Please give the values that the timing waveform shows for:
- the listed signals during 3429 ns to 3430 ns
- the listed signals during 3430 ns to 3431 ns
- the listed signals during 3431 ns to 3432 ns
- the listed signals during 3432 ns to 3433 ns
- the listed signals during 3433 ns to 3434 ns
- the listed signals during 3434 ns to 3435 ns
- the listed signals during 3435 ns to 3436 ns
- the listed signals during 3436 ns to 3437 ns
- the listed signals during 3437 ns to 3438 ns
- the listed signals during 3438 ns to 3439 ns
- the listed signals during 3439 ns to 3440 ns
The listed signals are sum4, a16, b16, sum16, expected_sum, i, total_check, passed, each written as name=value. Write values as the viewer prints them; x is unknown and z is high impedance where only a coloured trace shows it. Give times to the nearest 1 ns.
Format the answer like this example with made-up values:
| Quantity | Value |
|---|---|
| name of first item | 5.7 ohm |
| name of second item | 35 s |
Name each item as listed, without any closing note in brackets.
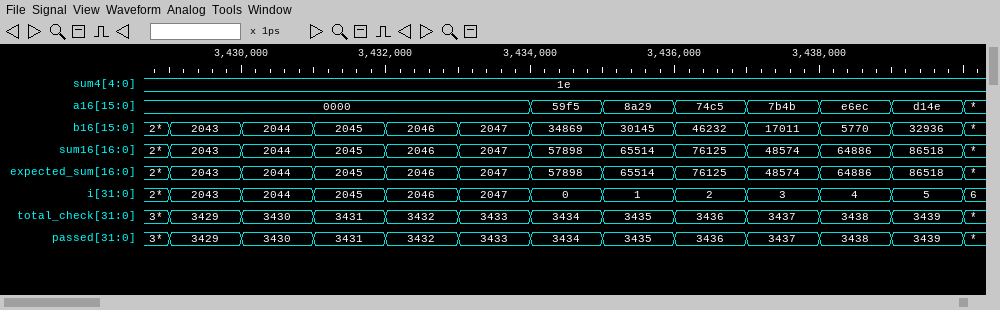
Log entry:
| Quantity | Value |
|---|---|
| the listed signals during 3429 ns to 3430 ns | sum4=1e, a16=0000, b16=2043, sum16=2043, expected_sum=2043, i=2043, total_check=3429, passed=3429 |
| the listed signals during 3430 ns to 3431 ns | sum4=1e, a16=0000, b16=2044, sum16=2044, expected_sum=2044, i=2044, total_check=3430, passed=3430 |
| the listed signals during 3431 ns to 3432 ns | sum4=1e, a16=0000, b16=2045, sum16=2045, expected_sum=2045, i=2045, total_check=3431, passed=3431 |
| the listed signals during 3432 ns to 3433 ns | sum4=1e, a16=0000, b16=2046, sum16=2046, expected_sum=2046, i=2046, total_check=3432, passed=3432 |
| the listed signals during 3433 ns to 3434 ns | sum4=1e, a16=0000, b16=2047, sum16=2047, expected_sum=2047, i=2047, total_check=3433, passed=3433 |
| the listed signals during 3434 ns to 3435 ns | sum4=1e, a16=59f5, b16=34869, sum16=57898, expected_sum=57898, i=0, total_check=3434, passed=3434 |
| the listed signals during 3435 ns to 3436 ns | sum4=1e, a16=8a29, b16=30145, sum16=65514, expected_sum=65514, i=1, total_check=3435, passed=3435 |
| the listed signals during 3436 ns to 3437 ns | sum4=1e, a16=74c5, b16=46232, sum16=76125, expected_sum=76125, i=2, total_check=3436, passed=3436 |
| the listed signals during 3437 ns to 3438 ns | sum4=1e, a16=7b4b, b16=17011, sum16=48574, expected_sum=48574, i=3, total_check=3437, passed=3437 |
| the listed signals during 3438 ns to 3439 ns | sum4=1e, a16=e6ec, b16=5770, sum16=64886, expected_sum=64886, i=4, total_check=3438, passed=3438 |
| the listed signals during 3439 ns to 3440 ns | sum4=1e, a16=d14e, b16=32936, sum16=86518, expected_sum=86518, i=5, total_check=3439, passed=3439 |
